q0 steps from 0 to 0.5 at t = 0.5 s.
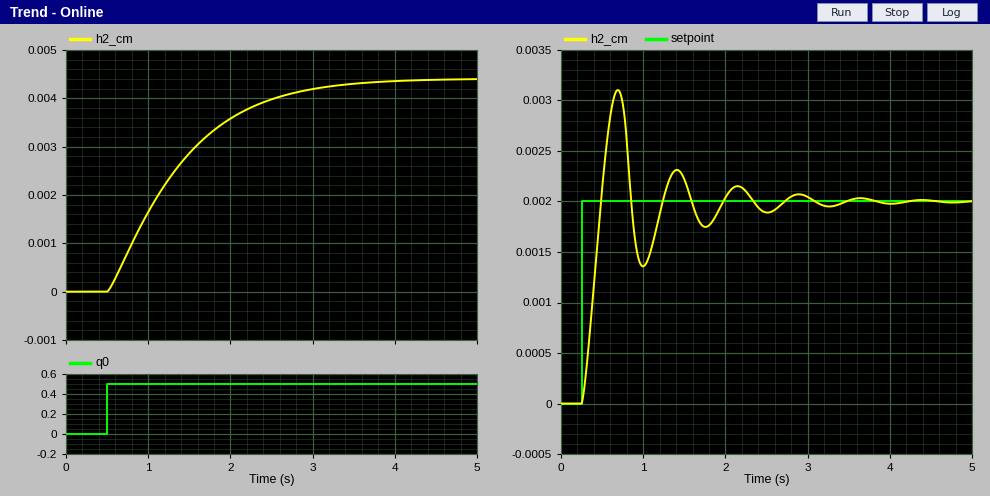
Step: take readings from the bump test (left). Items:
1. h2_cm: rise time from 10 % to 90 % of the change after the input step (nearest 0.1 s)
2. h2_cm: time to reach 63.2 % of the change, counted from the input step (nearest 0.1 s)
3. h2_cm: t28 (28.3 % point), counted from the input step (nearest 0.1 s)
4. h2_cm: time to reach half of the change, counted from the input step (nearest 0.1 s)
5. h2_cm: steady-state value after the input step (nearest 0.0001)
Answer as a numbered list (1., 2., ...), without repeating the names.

1. 1.8 s
2. 1.0 s
3. 0.4 s
4. 0.7 s
5. 0.0044
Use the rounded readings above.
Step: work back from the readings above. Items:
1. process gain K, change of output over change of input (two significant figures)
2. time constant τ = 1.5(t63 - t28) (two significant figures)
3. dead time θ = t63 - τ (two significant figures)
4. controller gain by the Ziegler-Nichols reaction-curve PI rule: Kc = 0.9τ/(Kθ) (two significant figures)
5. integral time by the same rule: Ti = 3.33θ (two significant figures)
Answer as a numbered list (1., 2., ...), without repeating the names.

1. 0.0088
2. 0.90 s
3. 0.10 s
4. 920
5. 0.33 s
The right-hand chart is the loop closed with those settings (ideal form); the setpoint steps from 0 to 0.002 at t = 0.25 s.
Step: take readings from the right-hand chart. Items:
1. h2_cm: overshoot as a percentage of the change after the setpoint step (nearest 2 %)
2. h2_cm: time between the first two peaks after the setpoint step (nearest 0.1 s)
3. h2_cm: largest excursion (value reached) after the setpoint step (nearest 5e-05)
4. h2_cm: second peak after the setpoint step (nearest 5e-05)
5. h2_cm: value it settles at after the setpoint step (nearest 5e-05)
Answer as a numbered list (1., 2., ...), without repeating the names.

1. 56 %
2. 0.7 s
3. 0.00310
4. 0.00230
5. 0.00200
